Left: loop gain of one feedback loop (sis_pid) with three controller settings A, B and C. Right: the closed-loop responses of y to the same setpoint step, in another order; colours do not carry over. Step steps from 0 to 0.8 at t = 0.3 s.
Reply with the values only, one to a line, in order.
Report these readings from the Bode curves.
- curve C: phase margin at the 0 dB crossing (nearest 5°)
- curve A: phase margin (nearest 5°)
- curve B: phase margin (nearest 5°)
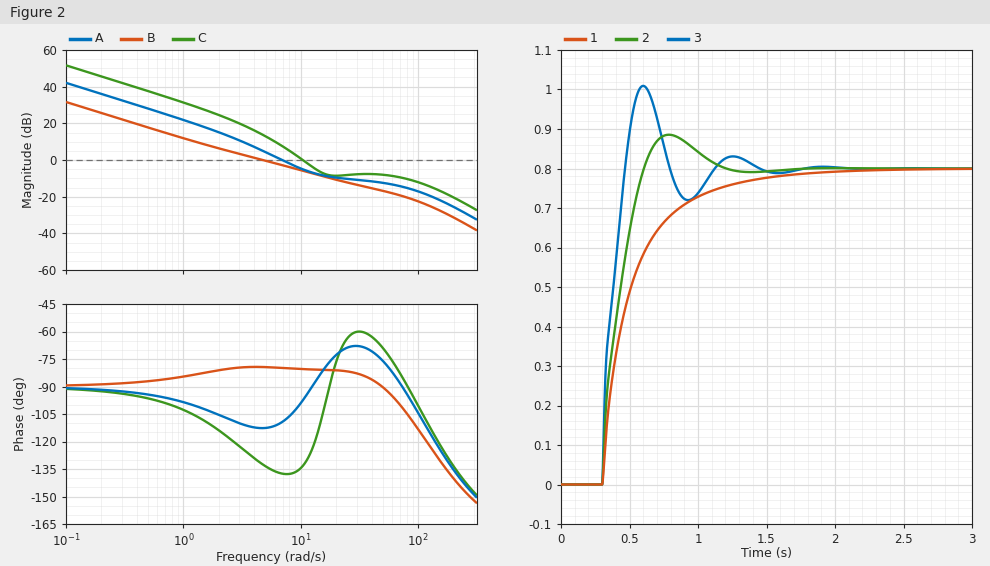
45°
70°
100°
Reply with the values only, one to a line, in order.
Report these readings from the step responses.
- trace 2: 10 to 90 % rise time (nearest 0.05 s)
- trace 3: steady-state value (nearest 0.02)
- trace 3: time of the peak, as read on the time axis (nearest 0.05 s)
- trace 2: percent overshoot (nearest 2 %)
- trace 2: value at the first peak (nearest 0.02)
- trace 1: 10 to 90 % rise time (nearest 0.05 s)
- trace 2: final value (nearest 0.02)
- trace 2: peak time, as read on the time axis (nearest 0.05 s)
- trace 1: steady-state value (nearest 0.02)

0.25 s
0.80
0.60 s
10 %
0.88
0.65 s
0.80
0.80 s
0.80
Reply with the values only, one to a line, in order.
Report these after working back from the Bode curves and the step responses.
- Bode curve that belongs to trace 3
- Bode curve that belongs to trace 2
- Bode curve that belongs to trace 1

C
A
B
